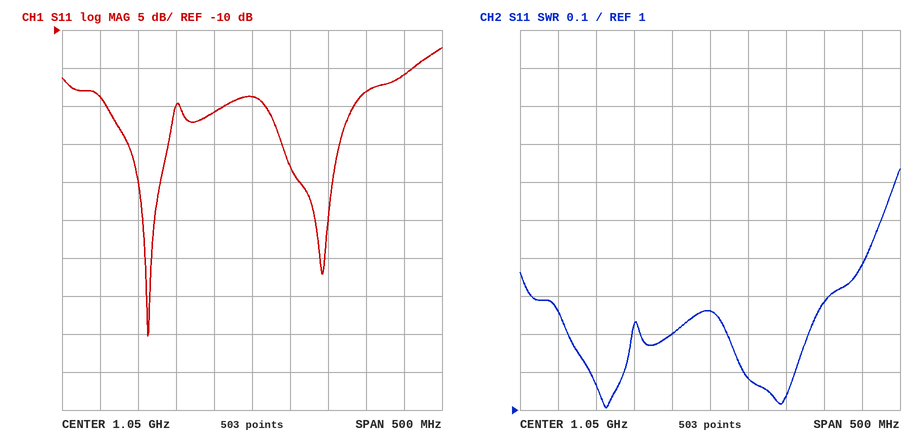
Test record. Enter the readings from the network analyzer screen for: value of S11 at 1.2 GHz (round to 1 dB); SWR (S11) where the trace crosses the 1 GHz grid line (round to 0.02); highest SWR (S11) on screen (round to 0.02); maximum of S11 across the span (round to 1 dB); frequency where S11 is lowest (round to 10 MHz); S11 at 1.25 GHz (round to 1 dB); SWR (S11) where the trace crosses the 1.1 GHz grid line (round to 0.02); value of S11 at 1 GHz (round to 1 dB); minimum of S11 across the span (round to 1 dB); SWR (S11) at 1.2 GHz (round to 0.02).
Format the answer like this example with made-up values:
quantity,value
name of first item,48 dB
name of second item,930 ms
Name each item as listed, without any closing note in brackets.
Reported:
quantity,value
value of S11 at 1.2 GHz,-18 dB
SWR (S11) where the trace crosses the 1 GHz grid line,1.20
highest SWR (S11) on screen,1.64
maximum of S11 across the span,-12 dB
frequency where S11 is lowest,910 MHz
S11 at 1.25 GHz,-16 dB
SWR (S11) where the trace crosses the 1.1 GHz grid line,1.08
value of S11 at 1 GHz,-21 dB
minimum of S11 across the span,-50 dB
SWR (S11) at 1.2 GHz,1.28
